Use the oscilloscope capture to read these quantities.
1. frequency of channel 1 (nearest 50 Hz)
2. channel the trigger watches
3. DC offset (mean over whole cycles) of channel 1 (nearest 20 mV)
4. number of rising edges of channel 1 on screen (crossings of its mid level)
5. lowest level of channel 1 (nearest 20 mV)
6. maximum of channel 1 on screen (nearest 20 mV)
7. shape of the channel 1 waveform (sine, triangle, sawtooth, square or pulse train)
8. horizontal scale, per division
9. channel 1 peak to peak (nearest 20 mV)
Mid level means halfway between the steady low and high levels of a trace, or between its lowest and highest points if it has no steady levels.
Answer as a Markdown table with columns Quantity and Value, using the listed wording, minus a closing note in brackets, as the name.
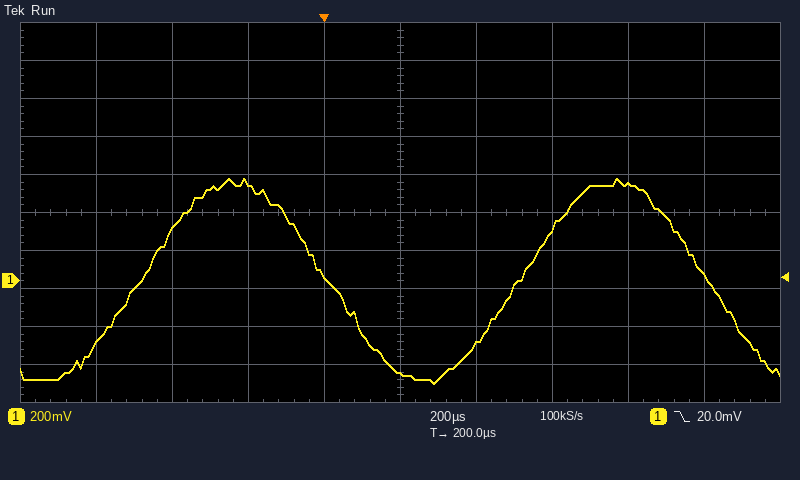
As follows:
| Quantity | Value |
|---|---|
| frequency of channel 1 | 1.00 kHz |
| channel the trigger watches | channel 1 |
| DC offset (mean over whole cycles) of channel 1 | 0 mV |
| number of rising edges of channel 1 on screen | 2 |
| lowest level of channel 1 | -540 mV |
| maximum of channel 1 on screen | 540 mV |
| shape of the channel 1 waveform | sine |
| horizontal scale, per division | 200 µs |
| channel 1 peak to peak | 1.08 V |
